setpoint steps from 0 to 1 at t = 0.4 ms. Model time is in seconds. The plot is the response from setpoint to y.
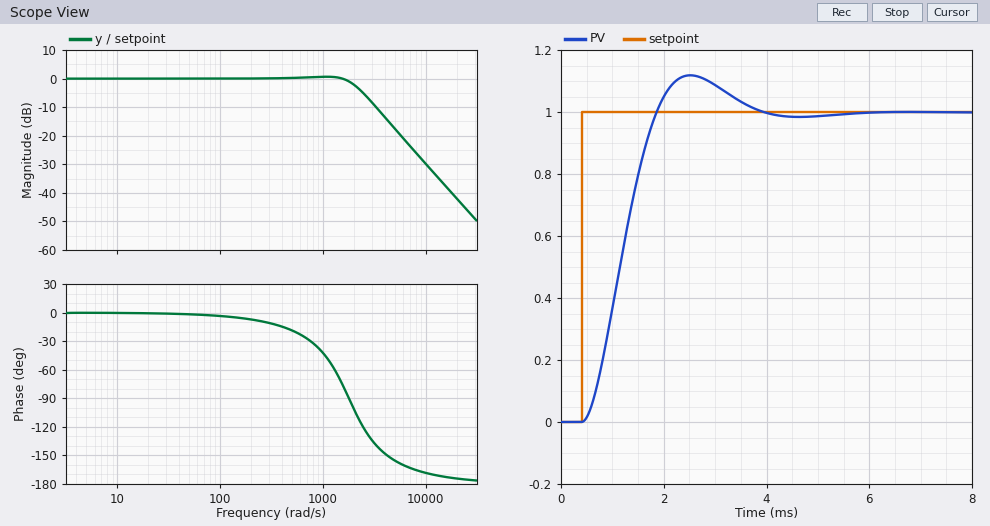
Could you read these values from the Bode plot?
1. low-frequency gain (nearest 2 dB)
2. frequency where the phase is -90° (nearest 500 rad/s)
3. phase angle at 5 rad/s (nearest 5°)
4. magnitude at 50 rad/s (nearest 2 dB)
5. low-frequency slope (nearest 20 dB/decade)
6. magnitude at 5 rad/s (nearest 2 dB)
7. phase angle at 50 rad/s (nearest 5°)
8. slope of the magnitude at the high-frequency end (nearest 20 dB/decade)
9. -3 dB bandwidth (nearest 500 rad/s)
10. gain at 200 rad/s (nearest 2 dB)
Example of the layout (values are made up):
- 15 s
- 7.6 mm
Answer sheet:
- 0 dB
- 2000 rad/s
- 0°
- 0 dB
- 0 dB/decade
- 0 dB
- 0°
- -40 dB/decade
- 2000 rad/s
- 0 dB
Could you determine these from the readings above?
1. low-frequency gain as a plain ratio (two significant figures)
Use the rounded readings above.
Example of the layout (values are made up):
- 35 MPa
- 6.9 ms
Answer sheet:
- 1.0
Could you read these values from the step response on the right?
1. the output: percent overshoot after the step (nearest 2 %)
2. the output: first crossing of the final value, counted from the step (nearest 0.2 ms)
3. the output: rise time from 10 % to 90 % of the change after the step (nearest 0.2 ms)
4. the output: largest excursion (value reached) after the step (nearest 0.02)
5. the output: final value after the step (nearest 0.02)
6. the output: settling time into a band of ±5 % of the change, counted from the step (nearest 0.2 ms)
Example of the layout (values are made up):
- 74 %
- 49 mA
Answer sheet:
- 12 %
- 1.4 ms
- 1.0 ms
- 1.12
- 1.00
- 3.0 ms
